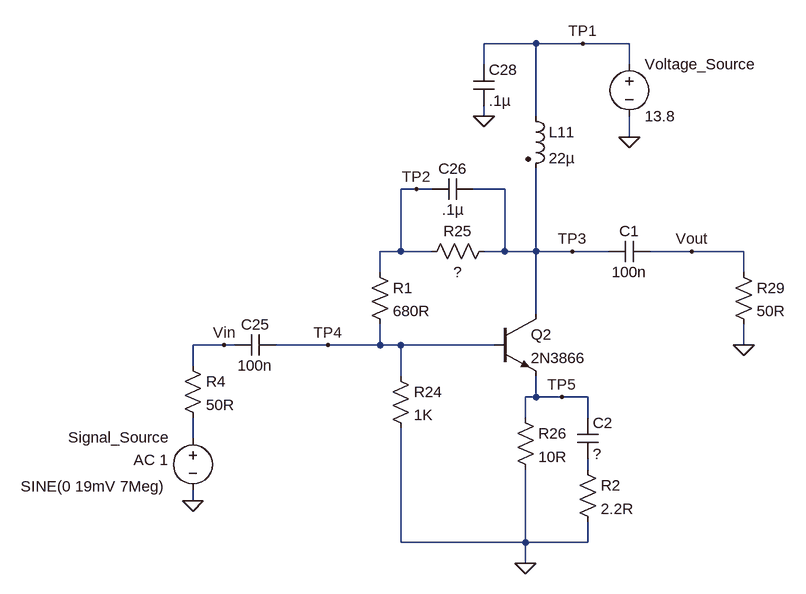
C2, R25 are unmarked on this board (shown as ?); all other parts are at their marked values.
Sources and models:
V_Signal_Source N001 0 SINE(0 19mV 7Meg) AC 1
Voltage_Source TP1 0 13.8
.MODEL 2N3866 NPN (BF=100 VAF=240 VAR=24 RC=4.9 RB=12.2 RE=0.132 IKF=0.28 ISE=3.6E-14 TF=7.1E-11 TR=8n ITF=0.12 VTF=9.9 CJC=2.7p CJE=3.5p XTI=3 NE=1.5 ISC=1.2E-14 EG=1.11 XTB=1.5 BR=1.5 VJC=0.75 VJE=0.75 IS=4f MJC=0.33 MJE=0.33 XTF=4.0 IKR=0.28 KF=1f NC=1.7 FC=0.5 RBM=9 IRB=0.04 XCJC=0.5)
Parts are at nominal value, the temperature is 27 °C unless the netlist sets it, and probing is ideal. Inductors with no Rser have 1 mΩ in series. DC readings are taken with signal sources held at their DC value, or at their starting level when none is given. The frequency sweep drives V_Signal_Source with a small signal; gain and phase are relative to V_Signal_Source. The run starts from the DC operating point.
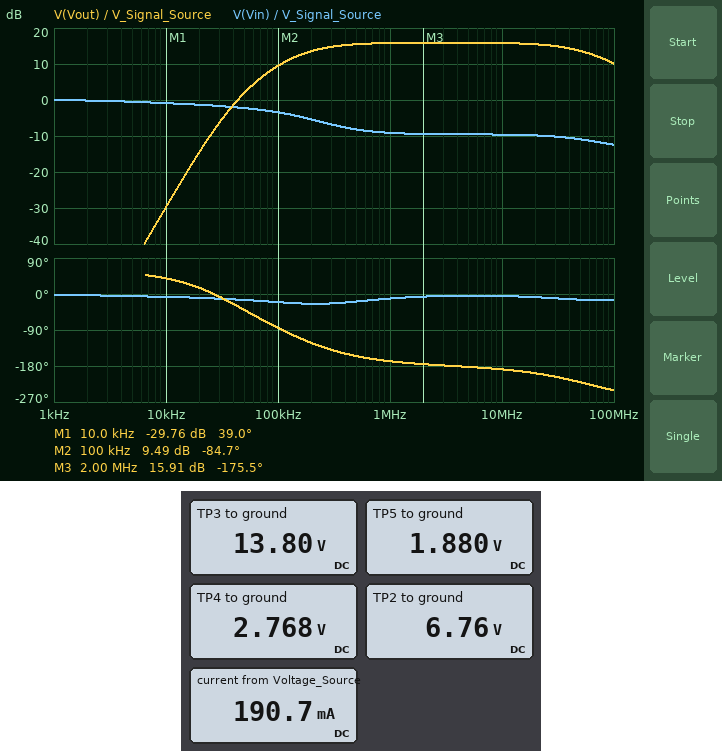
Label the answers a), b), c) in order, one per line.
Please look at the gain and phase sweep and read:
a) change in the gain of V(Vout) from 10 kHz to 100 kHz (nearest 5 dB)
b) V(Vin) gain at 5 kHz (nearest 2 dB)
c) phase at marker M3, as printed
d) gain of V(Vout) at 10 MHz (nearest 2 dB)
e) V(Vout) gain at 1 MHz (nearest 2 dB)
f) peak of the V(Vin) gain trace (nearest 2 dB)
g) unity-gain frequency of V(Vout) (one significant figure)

a) 40 dB
b) 0 dB
c) -175.5 deg
d) 16 dB
e) 16 dB
f) 0 dB
g) 40 kHz
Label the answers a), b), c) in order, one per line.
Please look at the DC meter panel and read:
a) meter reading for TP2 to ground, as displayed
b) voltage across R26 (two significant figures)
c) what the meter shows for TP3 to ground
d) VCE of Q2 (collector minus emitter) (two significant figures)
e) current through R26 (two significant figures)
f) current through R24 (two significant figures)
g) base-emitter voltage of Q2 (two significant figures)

a) 6.76 V
b) 1.9 V
c) 13.80 V
d) 12 V
e) 190 mA
f) 2.8 mA
g) 890 mV
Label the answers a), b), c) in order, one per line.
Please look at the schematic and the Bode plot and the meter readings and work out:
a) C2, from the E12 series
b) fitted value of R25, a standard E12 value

a) 1.5 µF
b) 1.2 kΩ
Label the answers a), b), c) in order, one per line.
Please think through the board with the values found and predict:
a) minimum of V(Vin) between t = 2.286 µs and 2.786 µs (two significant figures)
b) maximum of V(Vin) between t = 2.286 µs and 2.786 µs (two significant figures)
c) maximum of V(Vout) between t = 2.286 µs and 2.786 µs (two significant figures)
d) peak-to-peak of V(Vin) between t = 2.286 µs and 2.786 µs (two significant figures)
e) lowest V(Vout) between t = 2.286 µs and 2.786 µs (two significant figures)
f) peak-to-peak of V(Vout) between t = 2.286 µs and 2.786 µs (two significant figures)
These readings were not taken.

a) -6.3 mV
b) 6.3 mV
c) 120 mV
d) 13 mV
e) -120 mV
f) 240 mV
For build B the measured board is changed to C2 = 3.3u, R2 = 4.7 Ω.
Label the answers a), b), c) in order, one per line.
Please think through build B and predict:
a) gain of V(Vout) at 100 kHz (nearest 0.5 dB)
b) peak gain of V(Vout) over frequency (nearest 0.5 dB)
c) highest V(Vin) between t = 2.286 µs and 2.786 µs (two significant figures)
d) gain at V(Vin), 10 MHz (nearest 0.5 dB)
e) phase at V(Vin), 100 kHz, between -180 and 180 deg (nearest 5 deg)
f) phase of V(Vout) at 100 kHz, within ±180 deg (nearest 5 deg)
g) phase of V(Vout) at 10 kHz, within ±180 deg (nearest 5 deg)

a) 7.0 dB
b) 14.0 dB
c) 8.2 mV
d) -7.5 dB
e) -15 deg
f) -90 deg
g) 35 deg
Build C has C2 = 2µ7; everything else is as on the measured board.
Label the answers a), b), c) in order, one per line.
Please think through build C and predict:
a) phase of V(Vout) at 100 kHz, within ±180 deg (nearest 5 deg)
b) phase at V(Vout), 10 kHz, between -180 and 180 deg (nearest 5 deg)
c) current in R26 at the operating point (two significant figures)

a) -90 deg
b) 45 deg
c) 190 mA
